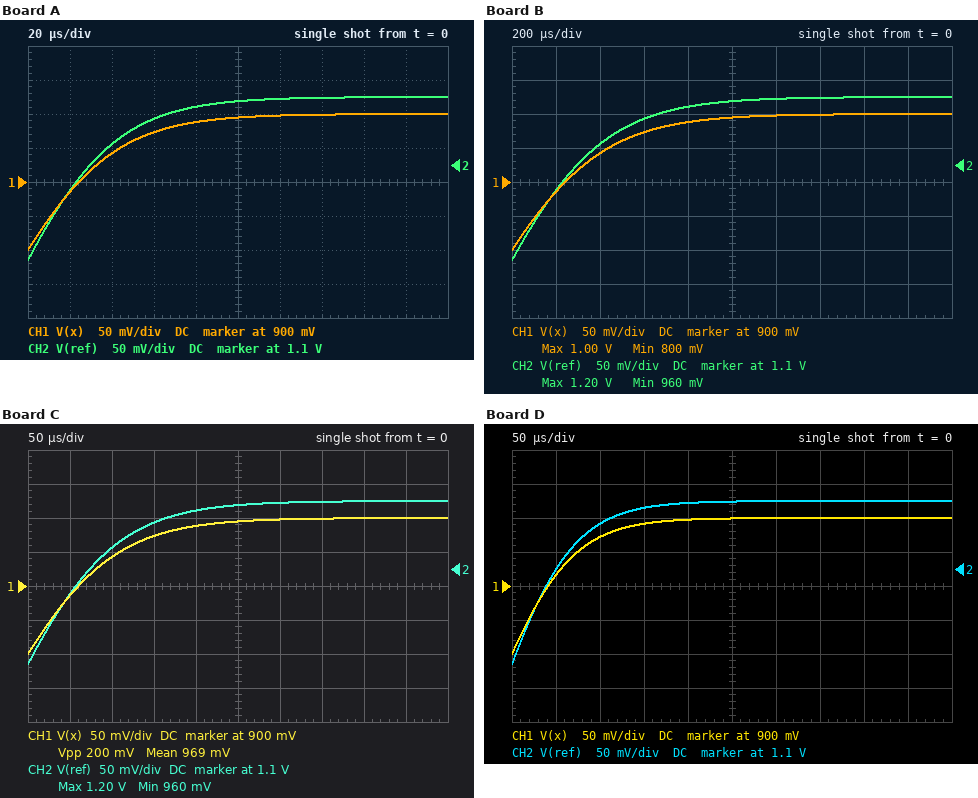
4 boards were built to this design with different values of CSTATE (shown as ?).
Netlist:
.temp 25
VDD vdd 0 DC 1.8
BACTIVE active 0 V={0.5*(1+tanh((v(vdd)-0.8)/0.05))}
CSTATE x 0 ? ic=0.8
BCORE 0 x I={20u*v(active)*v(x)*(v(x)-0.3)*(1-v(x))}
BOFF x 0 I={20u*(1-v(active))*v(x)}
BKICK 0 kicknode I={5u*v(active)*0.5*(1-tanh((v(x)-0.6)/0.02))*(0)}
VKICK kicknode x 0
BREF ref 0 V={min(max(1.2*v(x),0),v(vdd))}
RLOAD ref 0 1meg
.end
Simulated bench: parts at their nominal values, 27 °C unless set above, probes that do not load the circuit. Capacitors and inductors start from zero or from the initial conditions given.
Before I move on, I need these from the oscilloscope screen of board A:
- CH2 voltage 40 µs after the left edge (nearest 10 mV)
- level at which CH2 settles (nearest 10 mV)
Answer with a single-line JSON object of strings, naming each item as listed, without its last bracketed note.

{"CH2 voltage 40 µs after the left edge": "1.13 V", "level at which CH2 settles": "1.20 V"}
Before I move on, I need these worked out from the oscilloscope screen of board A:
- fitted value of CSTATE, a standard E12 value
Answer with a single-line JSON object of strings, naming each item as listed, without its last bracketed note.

{"fitted value of CSTATE, a standard E12 value": "330 pF"}
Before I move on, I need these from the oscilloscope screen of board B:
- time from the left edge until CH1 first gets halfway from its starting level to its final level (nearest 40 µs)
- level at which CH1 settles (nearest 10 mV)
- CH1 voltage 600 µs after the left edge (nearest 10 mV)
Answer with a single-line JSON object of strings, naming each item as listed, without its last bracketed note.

{"time from the left edge until CH1 first gets halfway from its starting level to its final level": "240 µs", "level at which CH1 settles": "1.00 V", "CH1 voltage 600 µs after the left edge": "970 mV"}
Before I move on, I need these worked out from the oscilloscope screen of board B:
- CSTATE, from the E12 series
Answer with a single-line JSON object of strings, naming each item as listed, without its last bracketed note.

{"CSTATE, from the E12 series": "3.3 nF"}
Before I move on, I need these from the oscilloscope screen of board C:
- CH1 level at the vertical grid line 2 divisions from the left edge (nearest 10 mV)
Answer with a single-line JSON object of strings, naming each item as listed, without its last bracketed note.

{"CH1 level at the vertical grid line 2 divisions from the left edge": "940 mV"}
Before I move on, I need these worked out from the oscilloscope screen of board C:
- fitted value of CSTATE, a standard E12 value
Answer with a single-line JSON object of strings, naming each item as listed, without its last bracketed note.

{"fitted value of CSTATE, a standard E12 value": "820 pF"}
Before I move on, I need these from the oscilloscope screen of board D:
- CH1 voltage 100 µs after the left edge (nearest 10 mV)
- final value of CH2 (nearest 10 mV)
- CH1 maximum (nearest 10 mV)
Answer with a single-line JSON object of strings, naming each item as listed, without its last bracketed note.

{"CH1 voltage 100 µs after the left edge": "970 mV", "final value of CH2": "1.20 V", "CH1 maximum": "1.00 V"}
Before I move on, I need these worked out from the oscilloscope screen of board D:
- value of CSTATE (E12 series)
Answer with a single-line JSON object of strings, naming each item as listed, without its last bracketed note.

{"value of CSTATE": "560 pF"}
